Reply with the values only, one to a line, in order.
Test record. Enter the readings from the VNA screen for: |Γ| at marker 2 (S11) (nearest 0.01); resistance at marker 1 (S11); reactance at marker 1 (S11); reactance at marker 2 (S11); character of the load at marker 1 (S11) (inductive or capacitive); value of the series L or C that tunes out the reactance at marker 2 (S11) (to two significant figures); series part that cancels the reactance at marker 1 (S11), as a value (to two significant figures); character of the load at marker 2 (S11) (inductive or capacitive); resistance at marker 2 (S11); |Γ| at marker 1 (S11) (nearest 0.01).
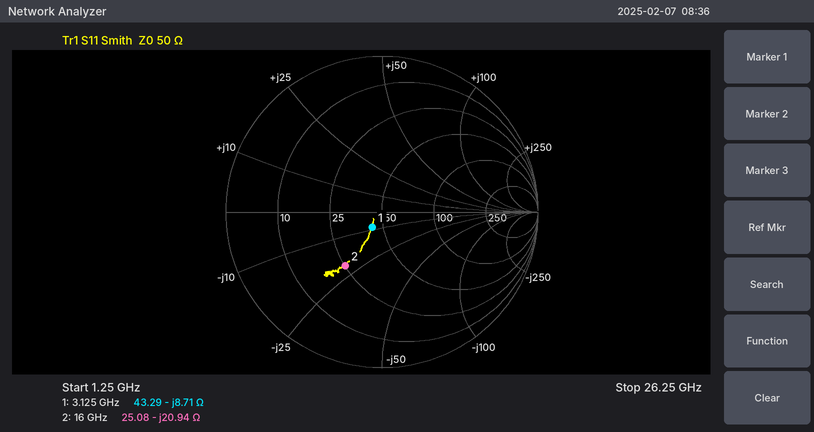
0.42
43.29 Ω
-8.71 Ω
-20.94 Ω
capacitive
210 pH
440 pH
capacitive
25.08 Ω
0.12
